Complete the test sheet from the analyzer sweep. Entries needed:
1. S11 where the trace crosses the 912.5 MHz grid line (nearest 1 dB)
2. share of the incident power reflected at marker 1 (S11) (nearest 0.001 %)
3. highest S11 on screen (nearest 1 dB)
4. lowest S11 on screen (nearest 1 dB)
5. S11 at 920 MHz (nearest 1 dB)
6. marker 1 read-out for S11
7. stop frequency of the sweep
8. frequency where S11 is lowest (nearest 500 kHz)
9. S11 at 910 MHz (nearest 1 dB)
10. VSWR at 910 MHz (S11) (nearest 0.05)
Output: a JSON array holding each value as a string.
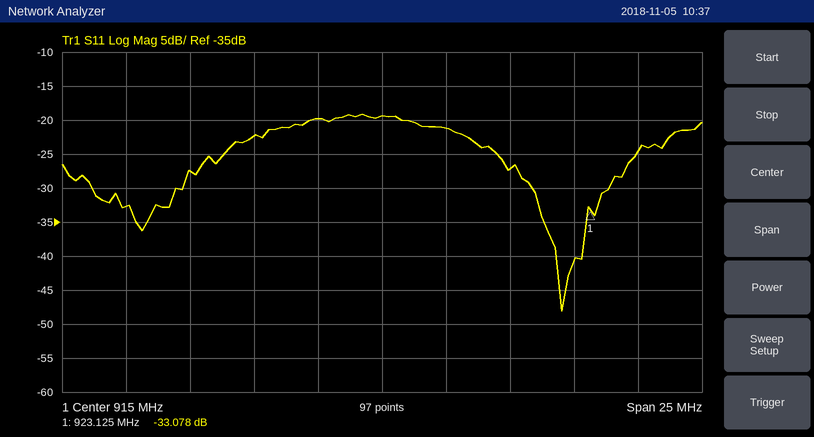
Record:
["-20 dB", "0.049 %", "-19 dB", "-48 dB", "-27 dB", "-33.078 dB", "927.5 MHz", "922.0 MHz", "-22 dB", "1.15"]
